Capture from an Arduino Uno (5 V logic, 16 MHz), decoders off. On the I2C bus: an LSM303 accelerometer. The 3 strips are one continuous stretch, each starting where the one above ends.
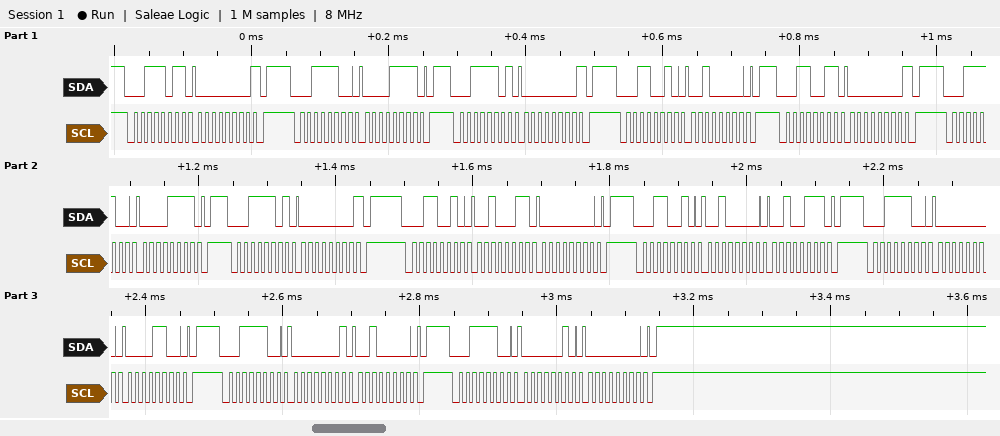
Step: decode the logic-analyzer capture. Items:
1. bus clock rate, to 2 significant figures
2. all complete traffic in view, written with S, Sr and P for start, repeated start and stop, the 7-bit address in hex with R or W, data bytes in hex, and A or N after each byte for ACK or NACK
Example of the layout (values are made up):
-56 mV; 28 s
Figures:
100 kHz; S 1DR A 00 N P S 1EW A 0F A P S 1ER A 00 N P S 19W A 20 A P S 19R A 00 N P S 1EW A 0F A P S 1ER A 00 N P S 19W A 23 A 00 A P S 19W A 20 A 27 A P S 1EW A 00 A 0C A P S 1EW A 01 A 20 A P S 1EW A 02 A 00 A P
